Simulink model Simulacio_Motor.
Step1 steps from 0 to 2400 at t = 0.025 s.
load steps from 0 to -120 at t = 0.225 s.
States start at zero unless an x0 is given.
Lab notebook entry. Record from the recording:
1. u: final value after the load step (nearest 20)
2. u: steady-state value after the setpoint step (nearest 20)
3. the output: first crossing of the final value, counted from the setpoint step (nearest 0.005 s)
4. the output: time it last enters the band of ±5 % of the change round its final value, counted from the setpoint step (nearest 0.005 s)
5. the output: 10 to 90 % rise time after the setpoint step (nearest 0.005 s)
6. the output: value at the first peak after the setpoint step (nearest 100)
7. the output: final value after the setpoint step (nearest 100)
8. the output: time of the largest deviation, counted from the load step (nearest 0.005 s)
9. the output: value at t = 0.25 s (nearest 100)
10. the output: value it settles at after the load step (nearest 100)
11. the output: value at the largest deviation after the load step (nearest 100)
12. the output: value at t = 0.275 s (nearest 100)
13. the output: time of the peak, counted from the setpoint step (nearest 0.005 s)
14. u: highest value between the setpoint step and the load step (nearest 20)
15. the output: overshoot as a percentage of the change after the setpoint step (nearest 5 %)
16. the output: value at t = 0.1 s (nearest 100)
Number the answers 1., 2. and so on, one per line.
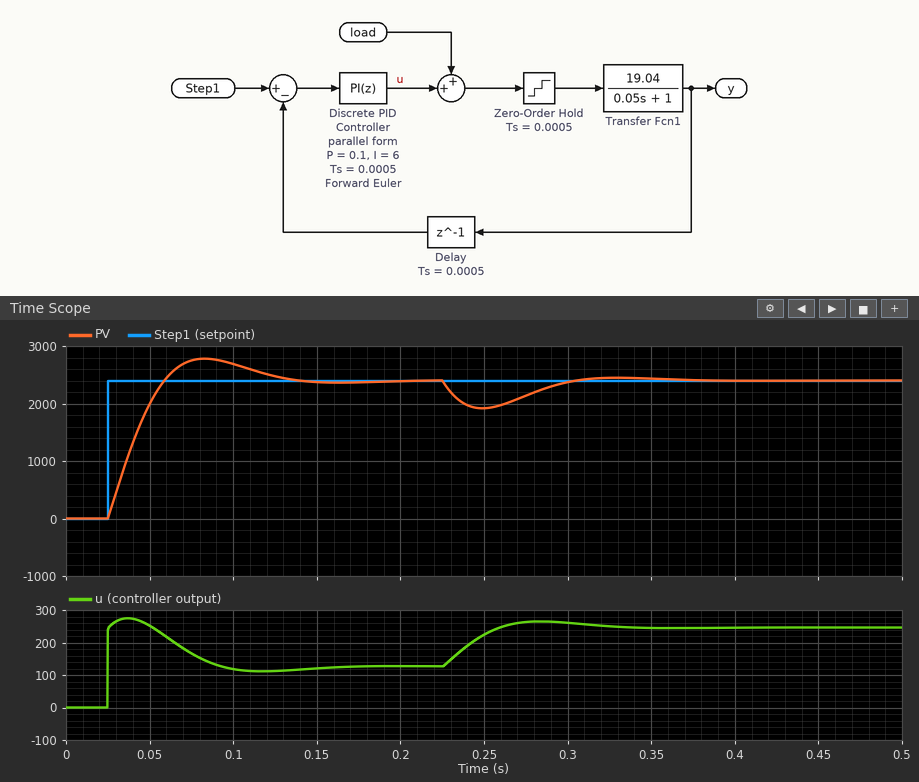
1. 240
2. 120
3. 0.035 s
4. 0.095 s
5. 0.025 s
6. 2800
7. 2400
8. 0.025 s
9. 1900
10. 2400
11. 1900
12. 2100
13. 0.060 s
14. 280
15. 15 %
16. 2700
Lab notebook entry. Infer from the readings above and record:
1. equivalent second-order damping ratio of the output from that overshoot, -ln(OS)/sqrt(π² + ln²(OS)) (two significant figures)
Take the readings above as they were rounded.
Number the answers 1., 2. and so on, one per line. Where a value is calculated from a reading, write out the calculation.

1. ln(0.15) = -1.897; 1.897 / sqrt(9.870 + 3.599) = 0.52
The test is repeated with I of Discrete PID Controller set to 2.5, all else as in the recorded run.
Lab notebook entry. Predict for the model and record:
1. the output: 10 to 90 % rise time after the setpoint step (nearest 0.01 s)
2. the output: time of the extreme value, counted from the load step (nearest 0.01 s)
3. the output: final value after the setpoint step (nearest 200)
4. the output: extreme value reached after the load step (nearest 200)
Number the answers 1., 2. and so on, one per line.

1. 0.05 s
2. 0.03 s
3. 2400
4. 1800
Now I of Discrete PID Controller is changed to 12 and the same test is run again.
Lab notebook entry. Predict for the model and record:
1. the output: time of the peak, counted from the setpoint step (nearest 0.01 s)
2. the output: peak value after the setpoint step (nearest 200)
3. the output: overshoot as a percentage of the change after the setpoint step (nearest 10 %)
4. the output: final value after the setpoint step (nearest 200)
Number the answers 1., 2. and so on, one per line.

1. 0.04 s
2. 3200
3. 30 %
4. 2400
